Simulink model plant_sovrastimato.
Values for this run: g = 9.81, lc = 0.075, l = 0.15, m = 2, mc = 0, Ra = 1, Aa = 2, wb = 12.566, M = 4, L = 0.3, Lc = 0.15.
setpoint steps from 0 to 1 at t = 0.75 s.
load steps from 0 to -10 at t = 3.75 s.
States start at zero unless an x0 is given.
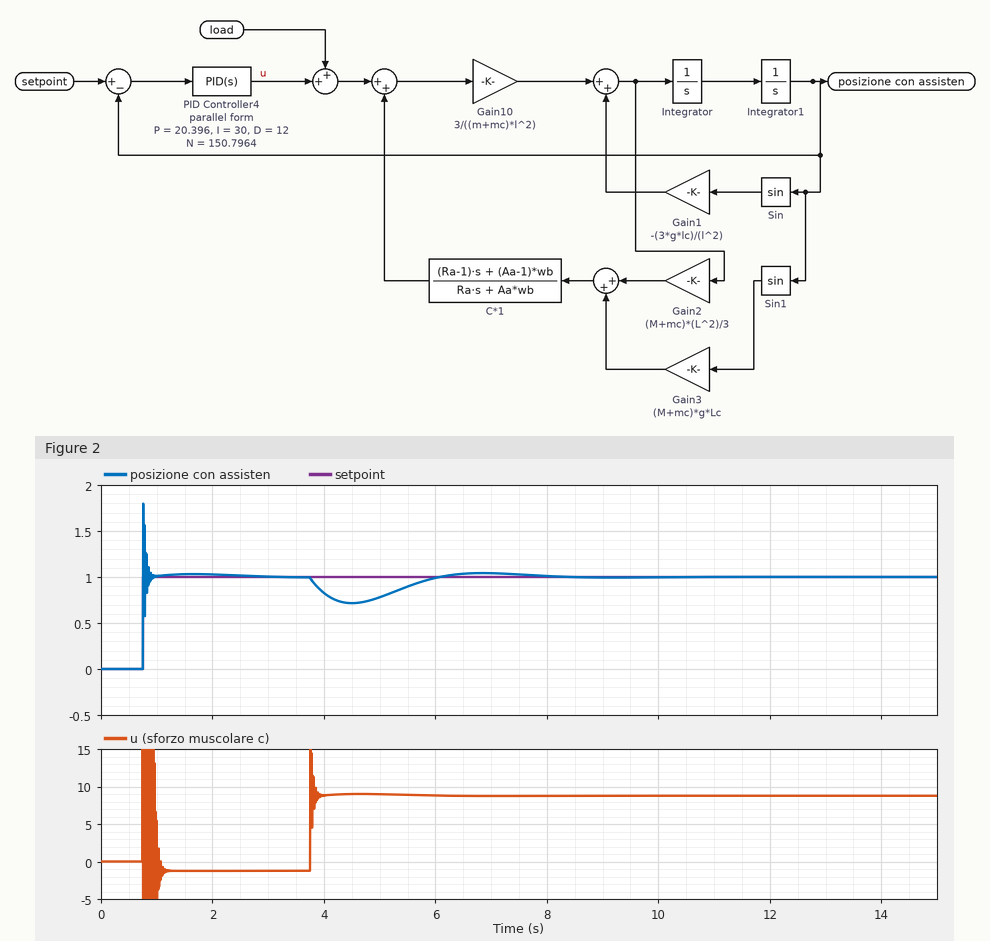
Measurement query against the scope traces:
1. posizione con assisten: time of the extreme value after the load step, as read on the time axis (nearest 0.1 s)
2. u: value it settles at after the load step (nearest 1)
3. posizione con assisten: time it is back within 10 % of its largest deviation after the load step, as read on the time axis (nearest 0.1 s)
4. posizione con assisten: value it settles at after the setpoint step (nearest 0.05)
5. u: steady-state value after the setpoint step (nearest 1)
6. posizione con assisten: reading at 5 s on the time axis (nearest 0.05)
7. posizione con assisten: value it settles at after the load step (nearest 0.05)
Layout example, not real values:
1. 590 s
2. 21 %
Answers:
1. 4.5 s
2. 9
3. 7.5 s
4. 1.00
5. -1
6. 0.80
7. 1.00
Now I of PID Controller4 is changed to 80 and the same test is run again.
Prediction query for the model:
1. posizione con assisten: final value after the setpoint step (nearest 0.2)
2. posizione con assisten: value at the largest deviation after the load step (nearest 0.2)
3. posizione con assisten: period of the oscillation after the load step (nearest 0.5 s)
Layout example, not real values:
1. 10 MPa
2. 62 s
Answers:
1. 1.0
2. 0.8
3. 2.5 s
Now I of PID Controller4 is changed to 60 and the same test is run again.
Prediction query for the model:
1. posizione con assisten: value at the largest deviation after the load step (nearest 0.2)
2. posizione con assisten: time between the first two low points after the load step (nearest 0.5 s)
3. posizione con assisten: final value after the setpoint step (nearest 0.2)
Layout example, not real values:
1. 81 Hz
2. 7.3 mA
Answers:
1. 0.8
2. 3.0 s
3. 1.0
